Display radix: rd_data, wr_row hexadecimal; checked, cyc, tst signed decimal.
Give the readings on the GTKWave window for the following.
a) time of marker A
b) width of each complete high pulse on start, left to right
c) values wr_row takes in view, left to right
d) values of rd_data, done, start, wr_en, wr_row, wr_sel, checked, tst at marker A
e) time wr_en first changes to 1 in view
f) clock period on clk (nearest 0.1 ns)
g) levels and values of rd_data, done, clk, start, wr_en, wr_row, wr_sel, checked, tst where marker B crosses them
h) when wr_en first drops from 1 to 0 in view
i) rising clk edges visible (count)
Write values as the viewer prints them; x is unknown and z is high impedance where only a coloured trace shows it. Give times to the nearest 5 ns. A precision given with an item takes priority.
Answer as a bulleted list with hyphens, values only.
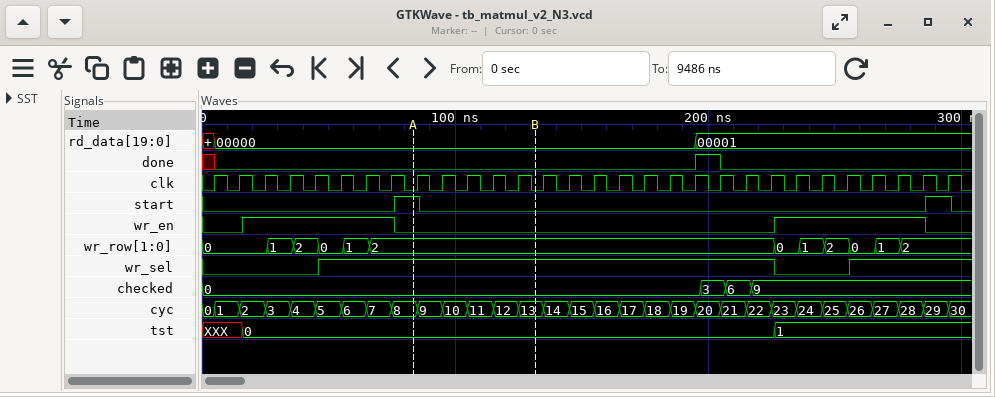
- 85 ns
- 10 ns, 10 ns
- 0, 1, 2, 0, 1, 2, 0, 1, 2, 0, 1, 2
- rd_data=00000, done=0, start=1, wr_en=0, wr_row=2, wr_sel=1, checked=0, tst=0
- 15 ns
- 10 ns
- rd_data=00000, done=0, clk=0, start=0, wr_en=0, wr_row=2, wr_sel=1, checked=0, tst=0
- 75 ns
- 30
